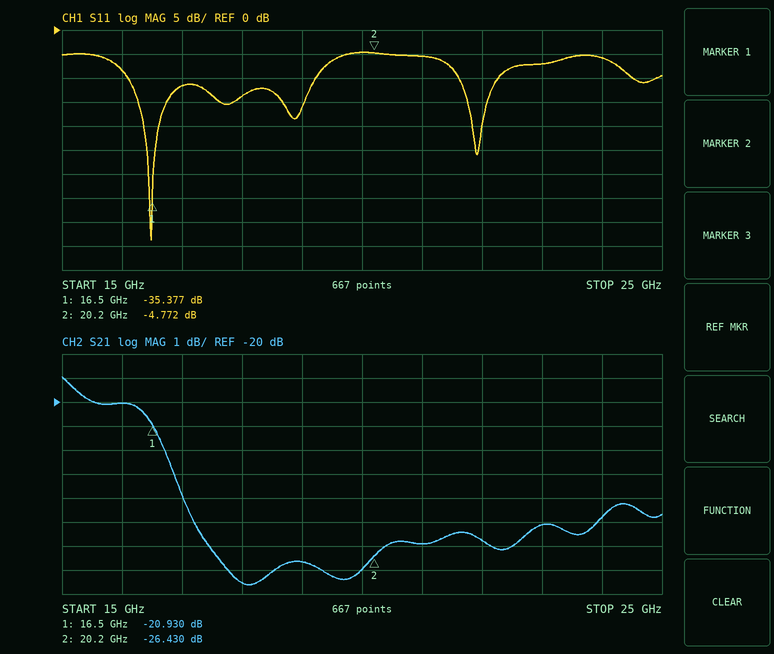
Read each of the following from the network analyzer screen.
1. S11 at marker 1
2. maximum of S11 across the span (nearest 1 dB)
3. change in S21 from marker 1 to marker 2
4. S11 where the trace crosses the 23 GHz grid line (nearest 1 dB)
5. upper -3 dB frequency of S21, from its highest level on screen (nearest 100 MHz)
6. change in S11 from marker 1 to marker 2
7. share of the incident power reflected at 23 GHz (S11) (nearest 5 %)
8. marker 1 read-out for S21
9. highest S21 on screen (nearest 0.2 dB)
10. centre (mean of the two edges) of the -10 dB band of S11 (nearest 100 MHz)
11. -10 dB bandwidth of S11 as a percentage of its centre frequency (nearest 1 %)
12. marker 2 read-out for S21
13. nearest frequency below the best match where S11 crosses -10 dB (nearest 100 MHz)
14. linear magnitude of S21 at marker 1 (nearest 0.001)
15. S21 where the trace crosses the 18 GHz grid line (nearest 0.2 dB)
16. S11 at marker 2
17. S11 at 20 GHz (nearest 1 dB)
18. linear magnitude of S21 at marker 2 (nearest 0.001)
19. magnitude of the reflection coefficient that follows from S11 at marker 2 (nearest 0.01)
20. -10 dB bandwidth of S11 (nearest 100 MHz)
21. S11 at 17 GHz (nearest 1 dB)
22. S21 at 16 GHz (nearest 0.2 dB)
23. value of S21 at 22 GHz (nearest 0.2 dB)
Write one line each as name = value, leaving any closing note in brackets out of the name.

S11 at marker 1 = -35.377 dB
maximum of S11 across the span = -5 dB
change in S21 from marker 1 to marker 2 = -5.500 dB
S11 where the trace crosses the 23 GHz grid line = -7 dB
upper -3 dB frequency of S21, from its highest level on screen = 16.7 GHz
change in S11 from marker 1 to marker 2 = 30.605 dB
share of the incident power reflected at 23 GHz (S11) = 20 %
marker 1 read-out for S21 = -20.930 dB
highest S21 on screen = -19.0 dB
centre (mean of the two edges) of the -10 dB band of S11 = 17.7 GHz
-10 dB bandwidth of S11 as a percentage of its centre frequency = 18 %
marker 2 read-out for S21 = -26.430 dB
nearest frequency below the best match where S11 crosses -10 dB = 16.1 GHz
linear magnitude of S21 at marker 1 = 0.090
S21 where the trace crosses the 18 GHz grid line = -27.6 dB
S11 at marker 2 = -4.772 dB
S11 at 20 GHz = -5 dB
linear magnitude of S21 at marker 2 = 0.048
magnitude of the reflection coefficient that follows from S11 at marker 2 = 0.58
-10 dB bandwidth of S11 = 3.1 GHz
S11 at 17 GHz = -12 dB
S21 at 16 GHz = -20.0 dB
value of S21 at 22 GHz = -25.8 dB
